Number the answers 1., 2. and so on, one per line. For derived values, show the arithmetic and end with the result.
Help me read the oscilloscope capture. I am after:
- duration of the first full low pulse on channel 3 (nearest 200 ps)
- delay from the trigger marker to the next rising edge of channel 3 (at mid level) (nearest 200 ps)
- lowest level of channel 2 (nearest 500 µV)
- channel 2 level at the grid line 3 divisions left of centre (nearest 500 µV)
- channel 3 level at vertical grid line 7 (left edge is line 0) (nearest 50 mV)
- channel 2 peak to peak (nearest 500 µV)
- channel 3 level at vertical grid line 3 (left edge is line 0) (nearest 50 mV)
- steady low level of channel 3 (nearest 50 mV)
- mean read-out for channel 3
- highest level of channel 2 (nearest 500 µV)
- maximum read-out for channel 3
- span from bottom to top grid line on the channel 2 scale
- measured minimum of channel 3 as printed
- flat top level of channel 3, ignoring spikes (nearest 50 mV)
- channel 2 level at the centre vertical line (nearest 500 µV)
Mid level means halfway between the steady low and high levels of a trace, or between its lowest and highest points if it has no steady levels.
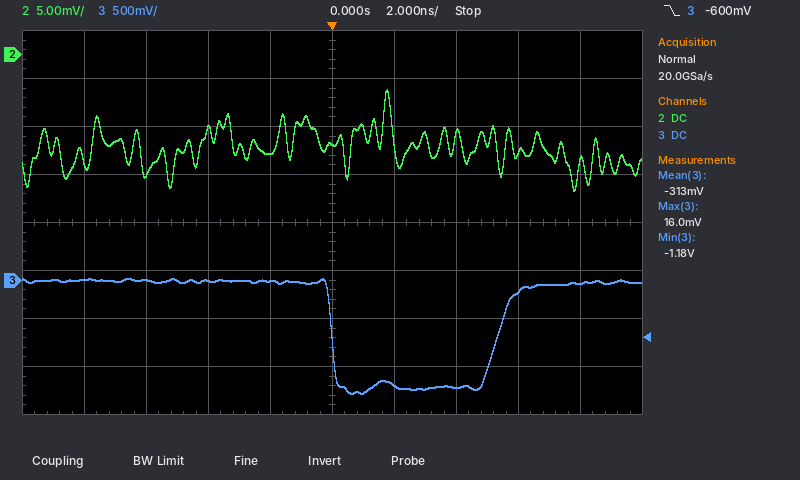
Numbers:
1. 5.4 ns
2. 5.4 ns
3. -14.0 mV
4. -12.5 mV
5. -1.10 V
6. -3.5 mV − (-14.0 mV) = 10.5 mV
7. 0 mV
8. -1.10 V
9. -313 mV
10. -3.5 mV
11. 16.0 mV
12. 40 mV
13. -1.18 V
14. 0 mV
15. -9.5 mV
